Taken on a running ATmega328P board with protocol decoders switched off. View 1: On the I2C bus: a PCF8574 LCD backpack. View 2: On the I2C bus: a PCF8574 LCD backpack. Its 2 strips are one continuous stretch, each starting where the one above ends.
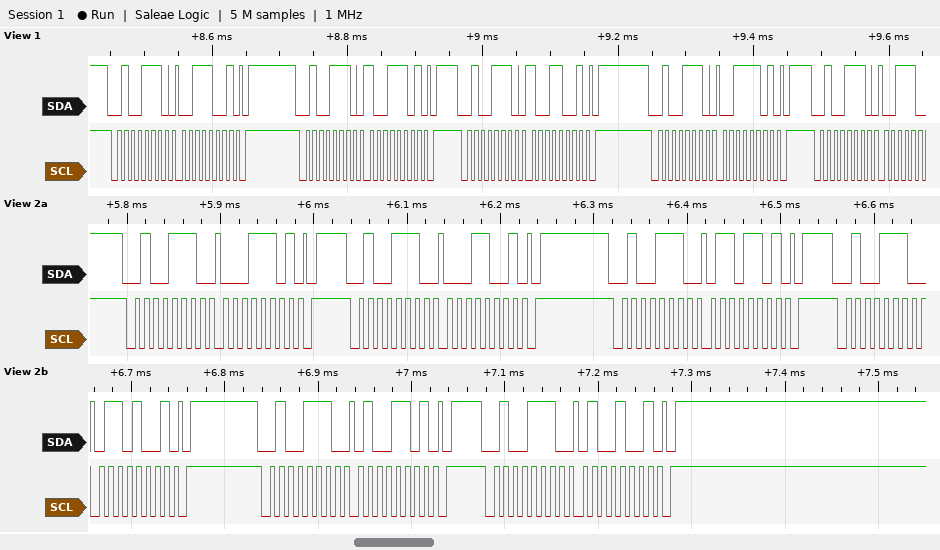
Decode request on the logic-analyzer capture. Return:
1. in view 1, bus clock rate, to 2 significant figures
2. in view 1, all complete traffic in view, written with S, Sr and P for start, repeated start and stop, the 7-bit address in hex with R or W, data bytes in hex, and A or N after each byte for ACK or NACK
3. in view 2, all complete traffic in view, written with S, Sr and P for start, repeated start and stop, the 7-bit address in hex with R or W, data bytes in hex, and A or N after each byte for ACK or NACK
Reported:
100 kHz
S 27W A 39 A P S 27W A 9D A P S 27W A 99 A P S 27W A 3D A P S 27W A
S 27W A 1D A P S 27W A 19 A P S 27W A 6D A P S 27W A 69 A P S 27W A 4D A P S 27W A 49 A P
